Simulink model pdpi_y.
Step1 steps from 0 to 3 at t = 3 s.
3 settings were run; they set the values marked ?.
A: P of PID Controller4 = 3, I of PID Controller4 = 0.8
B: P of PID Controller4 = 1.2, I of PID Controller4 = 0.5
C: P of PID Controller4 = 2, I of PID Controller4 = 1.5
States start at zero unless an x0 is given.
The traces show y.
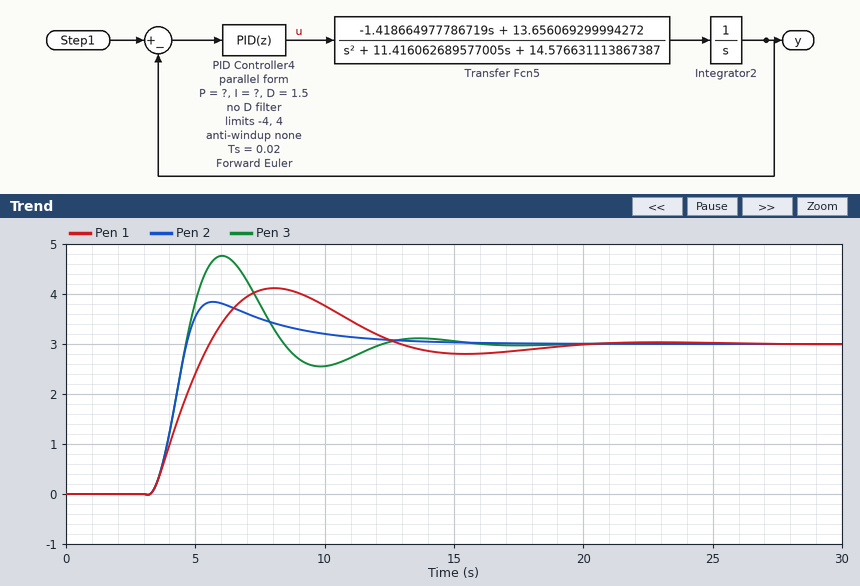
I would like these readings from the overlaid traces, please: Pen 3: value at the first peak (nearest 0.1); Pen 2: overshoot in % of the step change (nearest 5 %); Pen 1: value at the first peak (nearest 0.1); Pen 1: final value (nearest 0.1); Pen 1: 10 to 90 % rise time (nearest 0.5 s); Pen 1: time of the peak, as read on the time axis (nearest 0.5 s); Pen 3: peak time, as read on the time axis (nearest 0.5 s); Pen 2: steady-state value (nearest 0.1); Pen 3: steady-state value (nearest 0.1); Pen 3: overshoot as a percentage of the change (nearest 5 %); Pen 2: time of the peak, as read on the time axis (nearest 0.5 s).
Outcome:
4.8
30 %
4.1
3.0
1.5 s
8.0 s
6.0 s
3.0
3.0
60 %
5.5 s
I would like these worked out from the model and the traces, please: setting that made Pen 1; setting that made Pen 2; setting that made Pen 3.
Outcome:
B
A
C
